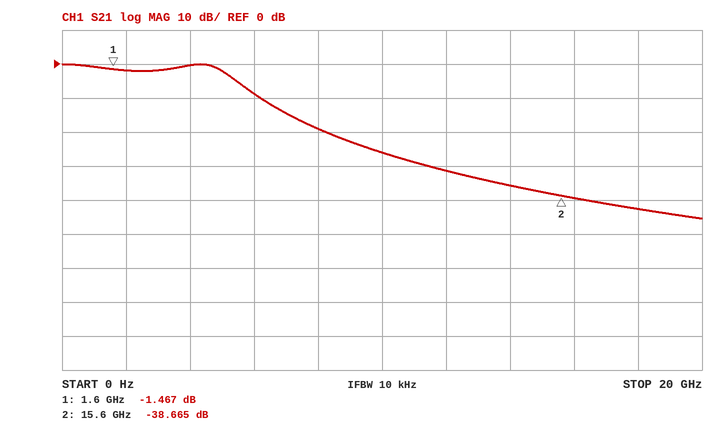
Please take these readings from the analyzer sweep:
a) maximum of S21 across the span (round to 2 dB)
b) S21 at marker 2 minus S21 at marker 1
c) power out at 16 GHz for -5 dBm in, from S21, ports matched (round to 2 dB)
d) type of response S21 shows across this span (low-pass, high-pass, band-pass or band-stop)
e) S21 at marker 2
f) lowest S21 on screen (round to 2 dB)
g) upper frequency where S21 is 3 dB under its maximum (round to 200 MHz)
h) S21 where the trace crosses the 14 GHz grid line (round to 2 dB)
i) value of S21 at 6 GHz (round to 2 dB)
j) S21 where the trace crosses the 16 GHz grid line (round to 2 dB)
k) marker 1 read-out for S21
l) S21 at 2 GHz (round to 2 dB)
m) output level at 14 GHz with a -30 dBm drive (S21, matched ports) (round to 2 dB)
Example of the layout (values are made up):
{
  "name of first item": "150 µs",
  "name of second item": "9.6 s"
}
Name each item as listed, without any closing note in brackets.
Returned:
{
  "maximum of S21 across the span": "0 dB",
  "S21 at marker 2 minus S21 at marker 1": "-37.198 dB",
  "power out at 16 GHz for -5 dBm in, from S21, ports matched": "-44 dBm",
  "type of response S21 shows across this span": "low-pass",
  "S21 at marker 2": "-38.665 dB",
  "lowest S21 on screen": "-46 dB",
  "upper frequency where S21 is 3 dB under its maximum": "5.2 GHz",
  "S21 where the trace crosses the 14 GHz grid line": "-36 dB",
  "value of S21 at 6 GHz": "-8 dB",
  "S21 where the trace crosses the 16 GHz grid line": "-40 dB",
  "marker 1 read-out for S21": "-1.467 dB",
  "S21 at 2 GHz": "-2 dB",
  "output level at 14 GHz with a -30 dBm drive (S21, matched ports)": "-66 dBm"
}
